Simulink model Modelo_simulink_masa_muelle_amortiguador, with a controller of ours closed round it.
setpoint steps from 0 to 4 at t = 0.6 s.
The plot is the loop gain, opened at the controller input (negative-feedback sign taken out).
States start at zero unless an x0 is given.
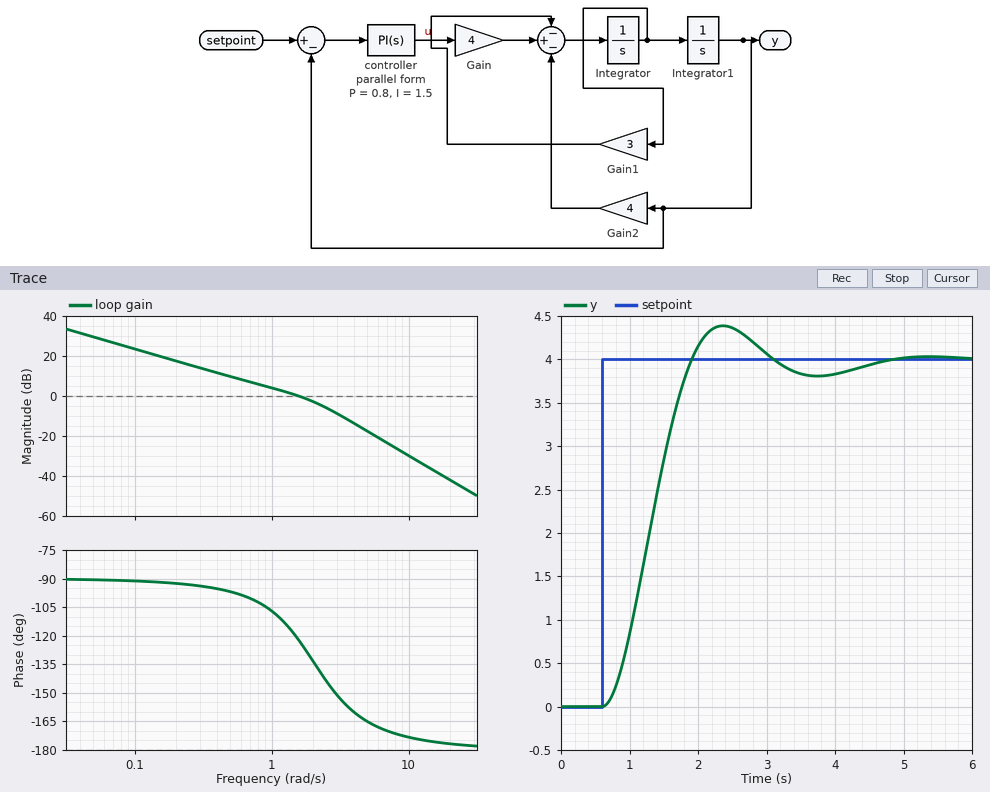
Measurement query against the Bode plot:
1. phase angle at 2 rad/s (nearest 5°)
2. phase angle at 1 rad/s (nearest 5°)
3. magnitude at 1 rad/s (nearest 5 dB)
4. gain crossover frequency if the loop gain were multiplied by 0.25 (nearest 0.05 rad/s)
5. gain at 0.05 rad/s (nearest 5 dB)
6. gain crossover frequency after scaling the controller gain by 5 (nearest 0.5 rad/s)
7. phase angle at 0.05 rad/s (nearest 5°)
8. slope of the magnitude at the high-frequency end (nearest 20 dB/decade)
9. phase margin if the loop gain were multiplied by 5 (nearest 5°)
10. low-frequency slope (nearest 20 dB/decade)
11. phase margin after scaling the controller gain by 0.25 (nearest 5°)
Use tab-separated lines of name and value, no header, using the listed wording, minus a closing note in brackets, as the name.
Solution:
phase angle at 2 rad/s	-135°
phase angle at 1 rad/s	-105°
magnitude at 1 rad/s	5 dB
gain crossover frequency if the loop gain were multiplied by 0.25	0.40 rad/s
gain at 0.05 rad/s	30 dB
gain crossover frequency after scaling the controller gain by 5	4.0 rad/s
phase angle at 0.05 rad/s	-90°
slope of the magnitude at the high-frequency end	-40 dB/decade
phase margin if the loop gain were multiplied by 5	20°
low-frequency slope	-20 dB/decade
phase margin after scaling the controller gain by 0.25	85°
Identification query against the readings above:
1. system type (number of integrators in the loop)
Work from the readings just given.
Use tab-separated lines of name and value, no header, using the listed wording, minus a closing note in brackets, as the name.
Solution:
system type	1
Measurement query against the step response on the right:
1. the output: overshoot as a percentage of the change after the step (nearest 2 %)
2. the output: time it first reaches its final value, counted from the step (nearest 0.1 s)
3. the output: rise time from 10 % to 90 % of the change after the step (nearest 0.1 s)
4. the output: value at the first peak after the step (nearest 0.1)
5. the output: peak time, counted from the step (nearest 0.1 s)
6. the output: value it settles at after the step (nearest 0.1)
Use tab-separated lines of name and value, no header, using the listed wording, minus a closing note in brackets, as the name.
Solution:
the output: overshoot as a percentage of the change after the step	10 %
the output: time it first reaches its final value, counted from the step	1.3 s
the output: rise time from 10 % to 90 % of the change after the step	0.9 s
the output: value at the first peak after the step	4.4
the output: peak time, counted from the step	1.8 s
the output: value it settles at after the step	4.0
